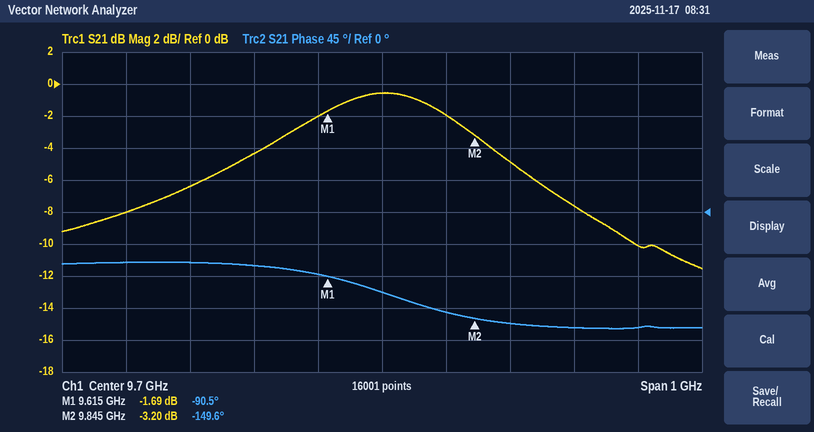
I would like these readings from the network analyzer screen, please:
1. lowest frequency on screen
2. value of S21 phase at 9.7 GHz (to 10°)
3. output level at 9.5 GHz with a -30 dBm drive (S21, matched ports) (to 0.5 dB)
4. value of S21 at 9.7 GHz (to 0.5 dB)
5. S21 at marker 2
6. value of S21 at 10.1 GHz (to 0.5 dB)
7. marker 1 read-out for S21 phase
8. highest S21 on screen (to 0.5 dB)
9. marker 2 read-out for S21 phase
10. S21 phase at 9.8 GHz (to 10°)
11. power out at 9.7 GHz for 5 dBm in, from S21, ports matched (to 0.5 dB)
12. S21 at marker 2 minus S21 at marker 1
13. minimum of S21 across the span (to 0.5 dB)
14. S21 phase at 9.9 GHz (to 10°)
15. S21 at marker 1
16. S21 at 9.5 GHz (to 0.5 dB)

9.2 GHz
-110°
-34.5 dBm
-0.5 dB
-3.20 dB
-10.0 dB
-90.5°
-0.5 dB
-149.6°
-140°
4.5 dBm
-1.51 dB
-11.5 dB
-160°
-1.69 dB
-4.5 dB
